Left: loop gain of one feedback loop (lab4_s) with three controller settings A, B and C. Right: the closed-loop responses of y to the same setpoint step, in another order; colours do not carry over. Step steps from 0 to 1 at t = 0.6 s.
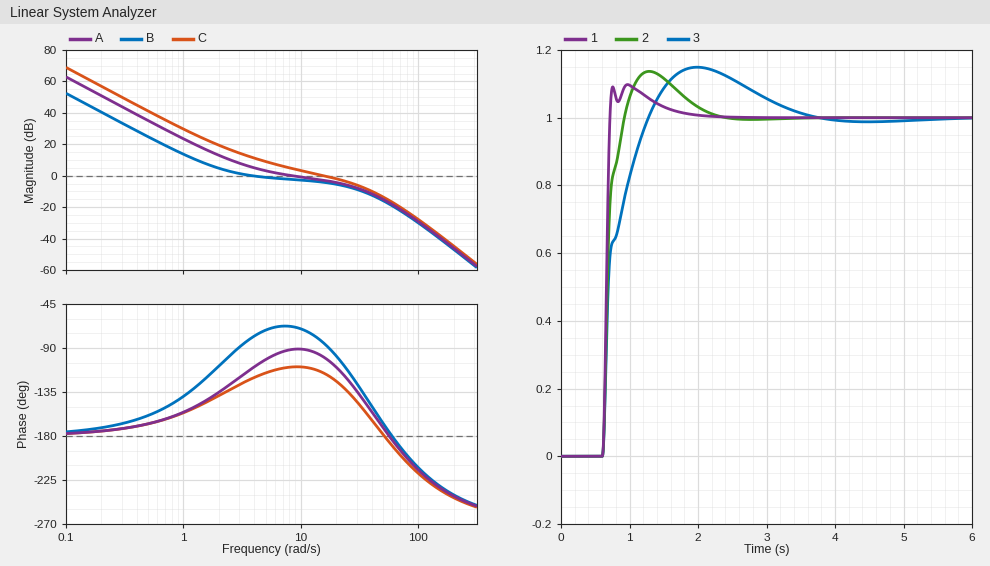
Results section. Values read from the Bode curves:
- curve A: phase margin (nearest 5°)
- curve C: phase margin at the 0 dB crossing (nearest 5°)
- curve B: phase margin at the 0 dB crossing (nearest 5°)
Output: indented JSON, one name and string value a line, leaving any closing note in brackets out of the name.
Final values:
{
  "curve A: phase margin": "90°",
  "curve C: phase margin at the 0 dB crossing": "65°",
  "curve B: phase margin at the 0 dB crossing": "100°"
}
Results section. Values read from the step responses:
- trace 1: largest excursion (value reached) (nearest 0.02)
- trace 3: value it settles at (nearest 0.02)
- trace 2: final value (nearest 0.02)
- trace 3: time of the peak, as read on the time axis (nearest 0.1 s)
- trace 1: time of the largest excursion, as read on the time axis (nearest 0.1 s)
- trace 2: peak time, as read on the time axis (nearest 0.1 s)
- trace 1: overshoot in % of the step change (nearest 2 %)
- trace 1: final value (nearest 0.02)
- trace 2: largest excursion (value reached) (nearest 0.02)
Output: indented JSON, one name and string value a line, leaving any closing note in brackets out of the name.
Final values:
{
  "trace 1: largest excursion (value reached)": "1.10",
  "trace 3: value it settles at": "1.00",
  "trace 2: final value": "1.00",
  "trace 3: time of the peak, as read on the time axis": "2.0 s",
  "trace 1: time of the largest excursion, as read on the time axis": "1.0 s",
  "trace 2: peak time, as read on the time axis": "1.3 s",
  "trace 1: overshoot in % of the step change": "10 %",
  "trace 1: final value": "1.00",
  "trace 2: largest excursion (value reached)": "1.14"
}
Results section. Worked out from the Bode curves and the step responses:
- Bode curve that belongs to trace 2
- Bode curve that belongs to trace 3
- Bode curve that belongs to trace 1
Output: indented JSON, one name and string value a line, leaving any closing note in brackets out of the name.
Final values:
{
  "Bode curve that belongs to trace 2": "A",
  "Bode curve that belongs to trace 3": "B",
  "Bode curve that belongs to trace 1": "C"
}
